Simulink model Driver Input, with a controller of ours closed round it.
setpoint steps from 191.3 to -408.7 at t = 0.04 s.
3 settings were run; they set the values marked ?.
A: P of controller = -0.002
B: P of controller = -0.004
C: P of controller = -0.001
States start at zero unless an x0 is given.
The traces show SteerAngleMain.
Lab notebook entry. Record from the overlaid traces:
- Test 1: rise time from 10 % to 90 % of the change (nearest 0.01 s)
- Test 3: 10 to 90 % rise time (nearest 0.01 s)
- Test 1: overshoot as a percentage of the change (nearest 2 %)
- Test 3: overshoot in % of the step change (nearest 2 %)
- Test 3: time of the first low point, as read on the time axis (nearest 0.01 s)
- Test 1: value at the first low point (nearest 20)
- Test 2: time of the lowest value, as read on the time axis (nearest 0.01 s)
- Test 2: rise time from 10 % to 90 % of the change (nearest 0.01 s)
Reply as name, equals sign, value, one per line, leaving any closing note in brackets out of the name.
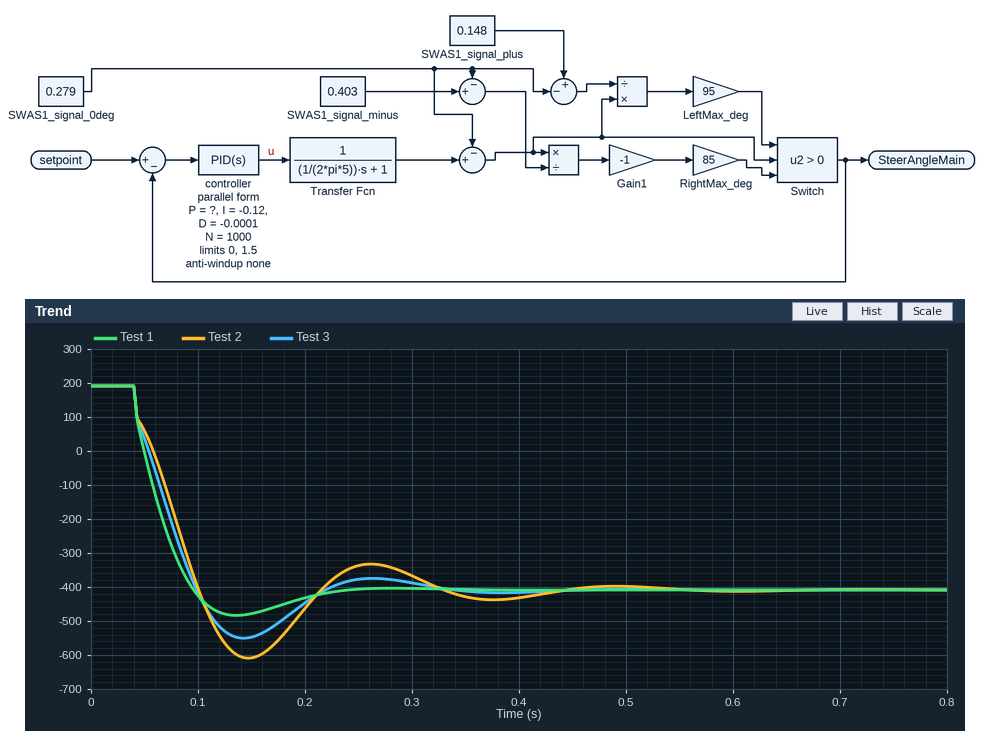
Test 1: rise time from 10 % to 90 % of the change = 0.04 s
Test 3: 10 to 90 % rise time = 0.05 s
Test 1: overshoot as a percentage of the change = 12 %
Test 3: overshoot in % of the step change = 24 %
Test 3: time of the first low point, as read on the time axis = 0.14 s
Test 1: value at the first low point = -480
Test 2: time of the lowest value, as read on the time axis = 0.15 s
Test 2: rise time from 10 % to 90 % of the change = 0.05 s
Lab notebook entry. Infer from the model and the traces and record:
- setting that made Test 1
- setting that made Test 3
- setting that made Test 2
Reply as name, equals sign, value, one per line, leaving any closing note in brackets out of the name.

setting that made Test 1 = B
setting that made Test 3 = A
setting that made Test 2 = C
